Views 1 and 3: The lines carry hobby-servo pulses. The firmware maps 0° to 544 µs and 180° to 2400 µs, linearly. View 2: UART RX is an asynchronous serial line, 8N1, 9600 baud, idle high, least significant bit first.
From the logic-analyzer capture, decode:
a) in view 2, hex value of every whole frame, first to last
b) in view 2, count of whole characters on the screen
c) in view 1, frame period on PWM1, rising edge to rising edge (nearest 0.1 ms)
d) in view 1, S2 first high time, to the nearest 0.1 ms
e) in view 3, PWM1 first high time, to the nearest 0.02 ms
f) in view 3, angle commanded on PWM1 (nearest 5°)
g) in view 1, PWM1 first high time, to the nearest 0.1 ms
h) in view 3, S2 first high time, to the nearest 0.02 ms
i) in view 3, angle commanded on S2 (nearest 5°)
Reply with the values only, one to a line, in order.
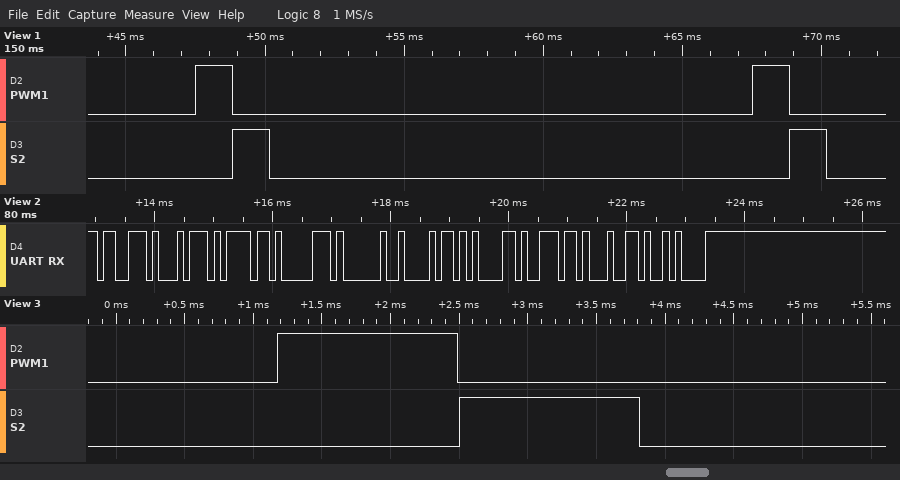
73 74 6F 70 20 68 61 6E 64 0A
10
20.0 ms
1.3 ms
1.32 ms
75°
1.3 ms
1.32 ms
75°
